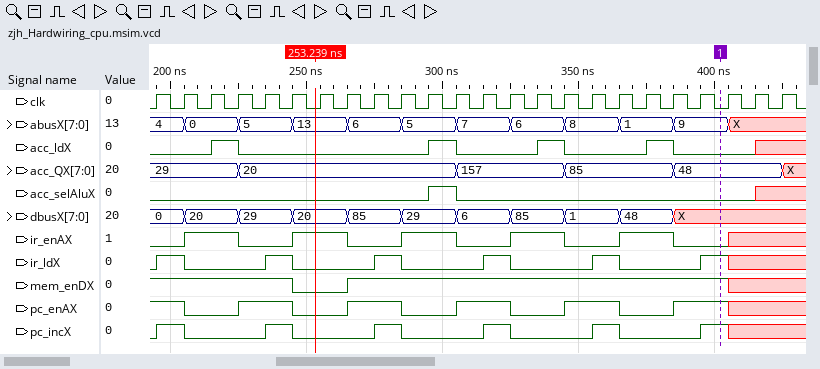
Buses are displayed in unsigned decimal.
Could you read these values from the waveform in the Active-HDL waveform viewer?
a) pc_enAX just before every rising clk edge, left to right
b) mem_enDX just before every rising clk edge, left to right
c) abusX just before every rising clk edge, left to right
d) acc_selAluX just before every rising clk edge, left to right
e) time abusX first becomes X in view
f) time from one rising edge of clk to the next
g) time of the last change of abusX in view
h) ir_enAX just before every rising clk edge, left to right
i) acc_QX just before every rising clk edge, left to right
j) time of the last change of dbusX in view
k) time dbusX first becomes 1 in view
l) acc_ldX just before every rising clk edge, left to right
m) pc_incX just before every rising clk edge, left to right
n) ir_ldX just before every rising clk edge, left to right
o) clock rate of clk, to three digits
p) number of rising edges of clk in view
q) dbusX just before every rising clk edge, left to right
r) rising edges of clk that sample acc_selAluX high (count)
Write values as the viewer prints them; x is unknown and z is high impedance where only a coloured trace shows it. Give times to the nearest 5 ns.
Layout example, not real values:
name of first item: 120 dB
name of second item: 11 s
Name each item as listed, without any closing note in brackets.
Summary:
pc_enAX just before every rising clk edge, left to right: 1 1 0 0 1 1 0 0 1 1 0 0 1 1 0 0 1 1 0 0 1 1 x x
mem_enDX just before every rising clk edge, left to right: 1 1 1 1 1 1 0 0 1 1 1 1 1 1 1 1 1 1 1 1 1 1 x x
abusX just before every rising clk edge, left to right: 4, 4, 0, 0, 5, 5, 13, 13, 6, 6, 5, 5, 7, 7, 6, 6, 8, 8, 1, 1, 9, 9, X, X
acc_selAluX just before every rising clk edge, left to right: 0 0 0 0 0 0 0 0 0 0 0 1 0 0 0 0 0 0 0 0 0 0 0 x
time abusX first becomes X in view: 405 ns
time from one rising edge of clk to the next: 10 ns
time of the last change of abusX in view: 405 ns
ir_enAX just before every rising clk edge, left to right: 0 0 1 1 0 0 1 1 0 0 1 1 0 0 1 1 0 0 1 1 0 0 x x
acc_QX just before every rising clk edge, left to right: 29, 29, 29, 29, 20, 20, 20, 20, 20, 20, 20, 20, 157, 157, 157, 157, 85, 85, 85, 85, 48, 48, 48, 48
time of the last change of dbusX in view: 385 ns
time dbusX first becomes 1 in view: 345 ns
acc_ldX just before every rising clk edge, left to right: 0 0 0 1 0 0 0 0 0 0 0 1 0 0 0 1 0 0 0 1 0 0 0 x
pc_incX just before every rising clk edge, left to right: 0 1 0 0 0 1 0 0 0 1 0 0 0 1 0 0 0 1 0 0 0 1 x x
ir_ldX just before every rising clk edge, left to right: 0 1 0 0 0 1 0 0 0 1 0 0 0 1 0 0 0 1 0 0 0 1 x x
clock rate of clk, to three digits: 100 MHz
number of rising edges of clk in view: 24
dbusX just before every rising clk edge, left to right: 0, 0, 20, 20, 29, 29, 20, 20, 85, 85, 29, 29, 6, 6, 85, 85, 1, 1, 48, 48, X, X, X, X
rising edges of clk that sample acc_selAluX high: 1
